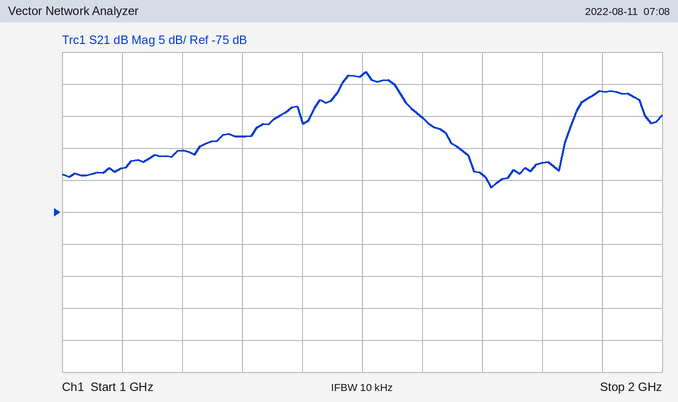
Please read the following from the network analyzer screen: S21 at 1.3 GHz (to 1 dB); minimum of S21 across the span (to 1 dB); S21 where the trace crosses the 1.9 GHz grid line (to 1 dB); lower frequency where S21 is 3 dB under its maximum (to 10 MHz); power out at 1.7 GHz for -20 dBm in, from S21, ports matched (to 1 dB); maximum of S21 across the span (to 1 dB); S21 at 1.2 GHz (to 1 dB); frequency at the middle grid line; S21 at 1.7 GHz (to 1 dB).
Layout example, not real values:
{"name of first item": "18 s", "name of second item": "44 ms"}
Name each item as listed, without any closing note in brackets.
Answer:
{"S21 at 1.3 GHz": "-63 dB", "minimum of S21 across the span": "-71 dB", "S21 where the trace crosses the 1.9 GHz grid line": "-56 dB", "lower frequency where S21 is 3 dB under its maximum": "1.46 GHz", "power out at 1.7 GHz for -20 dBm in, from S21, ports matched": "-89 dBm", "maximum of S21 across the span": "-53 dB", "S21 at 1.2 GHz": "-65 dB", "frequency at the middle grid line": "1.5 GHz", "S21 at 1.7 GHz": "-69 dB"}
